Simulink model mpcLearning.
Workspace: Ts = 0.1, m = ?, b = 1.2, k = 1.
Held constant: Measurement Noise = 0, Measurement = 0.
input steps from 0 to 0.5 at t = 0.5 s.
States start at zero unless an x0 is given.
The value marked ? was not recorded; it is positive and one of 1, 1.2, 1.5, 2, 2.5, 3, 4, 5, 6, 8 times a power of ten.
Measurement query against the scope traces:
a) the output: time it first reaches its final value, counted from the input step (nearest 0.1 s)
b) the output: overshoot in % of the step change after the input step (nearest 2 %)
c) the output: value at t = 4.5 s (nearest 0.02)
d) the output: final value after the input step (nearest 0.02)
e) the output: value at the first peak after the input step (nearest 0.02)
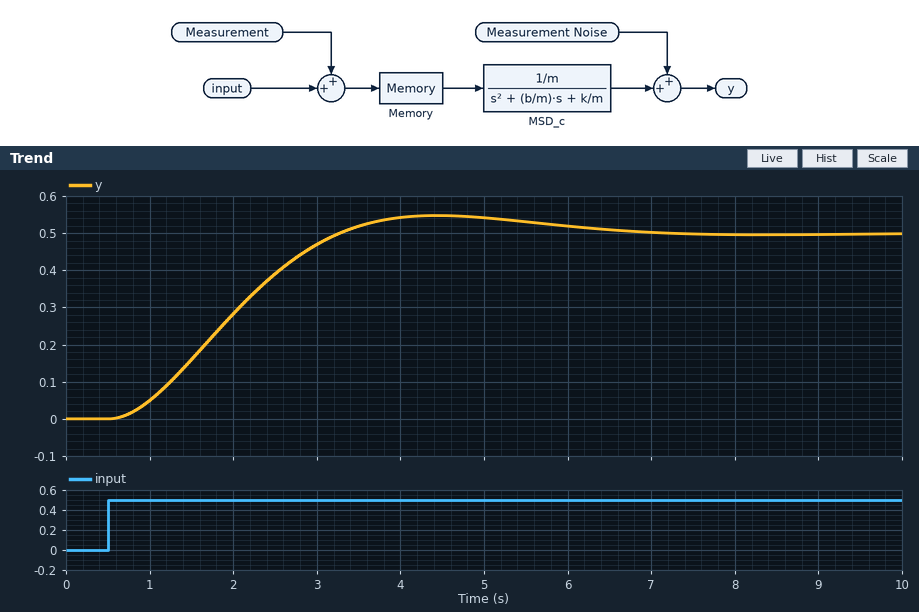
2.8 s
10 %
0.54
0.50
0.54
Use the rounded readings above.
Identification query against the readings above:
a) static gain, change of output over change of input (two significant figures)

1.0
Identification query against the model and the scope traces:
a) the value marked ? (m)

1
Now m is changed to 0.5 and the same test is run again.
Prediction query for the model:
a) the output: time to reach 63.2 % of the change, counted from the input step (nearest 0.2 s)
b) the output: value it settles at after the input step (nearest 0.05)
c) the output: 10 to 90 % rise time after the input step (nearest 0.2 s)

1.4 s
0.50
1.8 s
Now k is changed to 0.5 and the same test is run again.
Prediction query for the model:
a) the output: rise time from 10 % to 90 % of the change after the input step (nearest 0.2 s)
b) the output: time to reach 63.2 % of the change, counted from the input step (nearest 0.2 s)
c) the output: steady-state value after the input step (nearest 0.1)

3.8 s
2.8 s
1.0
